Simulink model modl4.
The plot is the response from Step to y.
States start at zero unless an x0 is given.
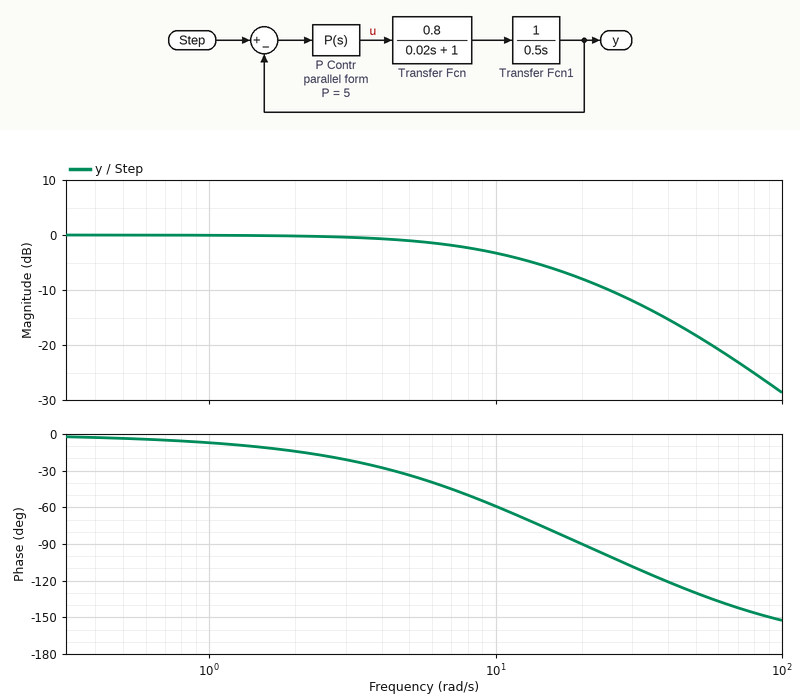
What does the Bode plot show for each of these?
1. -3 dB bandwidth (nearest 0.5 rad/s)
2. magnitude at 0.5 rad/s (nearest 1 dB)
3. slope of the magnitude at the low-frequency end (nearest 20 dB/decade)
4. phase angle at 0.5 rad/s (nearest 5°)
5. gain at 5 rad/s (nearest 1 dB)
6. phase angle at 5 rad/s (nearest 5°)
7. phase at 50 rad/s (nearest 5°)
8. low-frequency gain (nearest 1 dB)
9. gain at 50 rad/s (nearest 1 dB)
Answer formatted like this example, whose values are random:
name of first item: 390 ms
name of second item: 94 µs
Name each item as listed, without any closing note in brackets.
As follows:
-3 dB bandwidth: 9.5 rad/s
magnitude at 0.5 rad/s: 0 dB
slope of the magnitude at the low-frequency end: 0 dB/decade
phase angle at 0.5 rad/s: -5°
gain at 5 rad/s: -1 dB
phase angle at 5 rad/s: -35°
phase at 50 rad/s: -130°
low-frequency gain: 0 dB
gain at 50 rad/s: -18 dB
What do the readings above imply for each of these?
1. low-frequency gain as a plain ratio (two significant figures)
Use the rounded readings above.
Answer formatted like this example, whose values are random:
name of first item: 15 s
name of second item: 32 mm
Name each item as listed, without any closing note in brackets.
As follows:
low-frequency gain as a plain ratio: 1.0
